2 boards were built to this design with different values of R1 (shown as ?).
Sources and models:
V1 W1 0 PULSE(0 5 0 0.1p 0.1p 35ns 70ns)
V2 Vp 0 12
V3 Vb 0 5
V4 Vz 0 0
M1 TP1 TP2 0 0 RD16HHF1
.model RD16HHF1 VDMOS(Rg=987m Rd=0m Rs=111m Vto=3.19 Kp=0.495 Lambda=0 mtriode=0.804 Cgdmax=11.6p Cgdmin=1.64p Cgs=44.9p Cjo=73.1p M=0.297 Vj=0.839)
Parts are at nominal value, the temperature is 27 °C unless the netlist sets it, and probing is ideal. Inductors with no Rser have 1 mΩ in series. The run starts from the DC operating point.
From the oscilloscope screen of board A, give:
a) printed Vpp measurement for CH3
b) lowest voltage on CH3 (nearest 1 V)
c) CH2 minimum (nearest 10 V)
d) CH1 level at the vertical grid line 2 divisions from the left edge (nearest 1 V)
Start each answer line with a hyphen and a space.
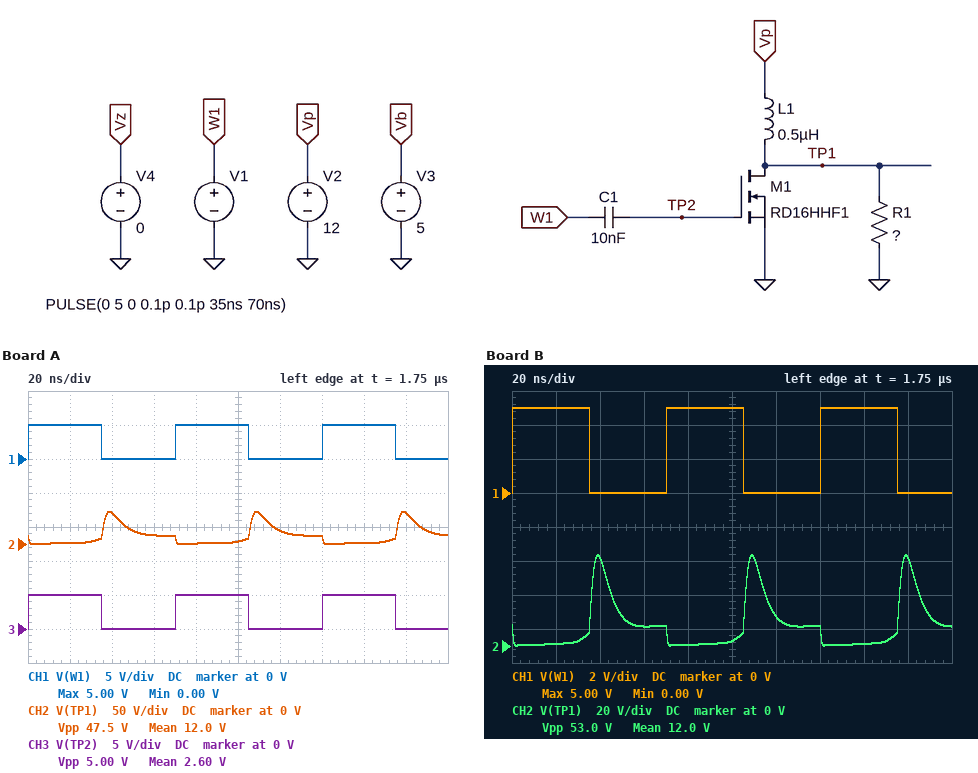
- 5.00 V
- 0 V
- 0 V
- 0 V
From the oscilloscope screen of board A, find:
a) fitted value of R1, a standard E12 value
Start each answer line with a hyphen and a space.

- 68 Ω
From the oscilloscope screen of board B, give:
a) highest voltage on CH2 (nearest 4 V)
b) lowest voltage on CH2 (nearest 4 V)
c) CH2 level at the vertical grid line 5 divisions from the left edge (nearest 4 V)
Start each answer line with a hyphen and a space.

- 52 V
- 0 V
- 4 V
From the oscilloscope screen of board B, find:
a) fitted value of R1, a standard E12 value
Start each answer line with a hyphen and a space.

- 82 Ω
